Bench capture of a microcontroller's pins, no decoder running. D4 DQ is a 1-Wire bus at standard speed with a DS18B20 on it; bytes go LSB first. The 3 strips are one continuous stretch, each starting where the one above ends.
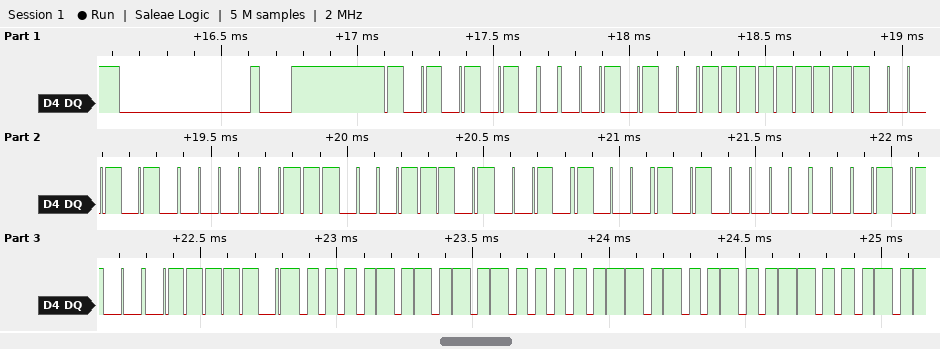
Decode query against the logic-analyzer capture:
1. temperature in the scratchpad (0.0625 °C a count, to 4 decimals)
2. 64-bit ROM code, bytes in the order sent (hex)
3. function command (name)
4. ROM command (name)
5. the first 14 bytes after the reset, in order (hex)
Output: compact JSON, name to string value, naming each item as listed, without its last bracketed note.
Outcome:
{"temperature in the scratchpad": "85.0000 °C", "64-bit ROM code, bytes in the order sent": "28 FF 51 E0 B8 14 05 28", "function command": "Read Scratchpad", "ROM command": "Match ROM", "the first 14 bytes after the reset, in order": "55 28 FF 51 E0 B8 14 05 28 BE 50 05 4B 46"}
